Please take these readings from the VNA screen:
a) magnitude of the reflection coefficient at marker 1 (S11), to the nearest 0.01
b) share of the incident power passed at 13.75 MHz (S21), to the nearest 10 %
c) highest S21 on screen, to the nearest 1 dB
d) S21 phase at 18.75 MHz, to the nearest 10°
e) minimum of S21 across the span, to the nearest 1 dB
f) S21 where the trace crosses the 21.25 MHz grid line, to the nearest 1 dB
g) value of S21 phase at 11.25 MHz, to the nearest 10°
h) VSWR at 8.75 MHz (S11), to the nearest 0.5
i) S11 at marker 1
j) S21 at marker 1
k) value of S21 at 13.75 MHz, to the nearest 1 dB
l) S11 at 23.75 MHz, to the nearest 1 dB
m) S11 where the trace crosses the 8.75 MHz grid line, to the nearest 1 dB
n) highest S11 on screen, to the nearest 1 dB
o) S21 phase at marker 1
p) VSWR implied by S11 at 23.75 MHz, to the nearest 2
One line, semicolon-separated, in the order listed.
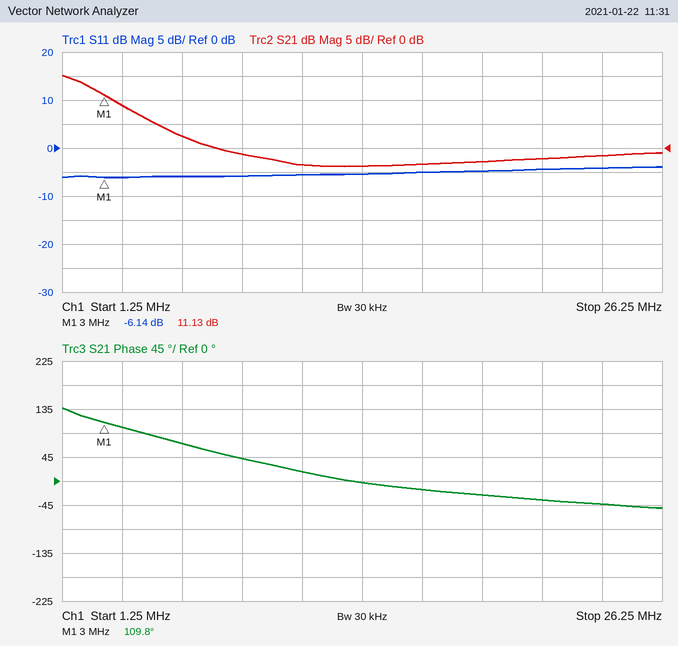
0.49; 40 %; 15 dB; -30°; -4 dB; -2 dB; 20°; 3.0; -6.14 dB; 11.13 dB; -4 dB; -4 dB; -6 dB; -4 dB; 109.8°; 4
